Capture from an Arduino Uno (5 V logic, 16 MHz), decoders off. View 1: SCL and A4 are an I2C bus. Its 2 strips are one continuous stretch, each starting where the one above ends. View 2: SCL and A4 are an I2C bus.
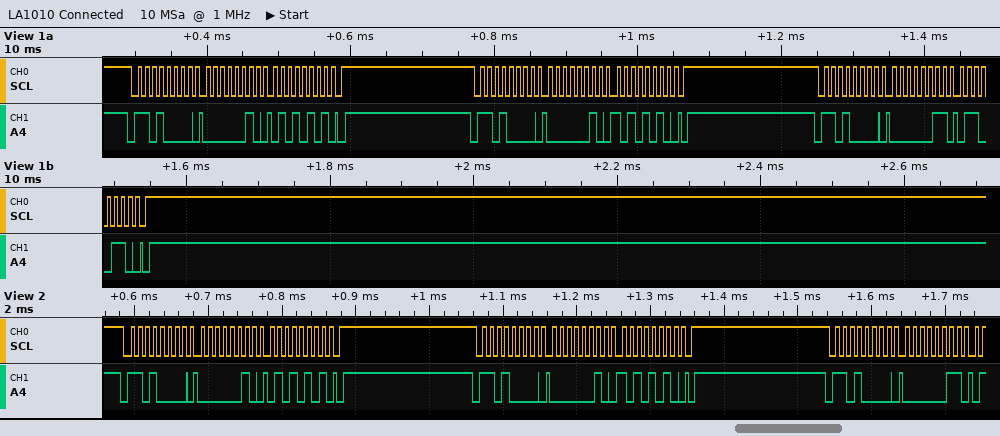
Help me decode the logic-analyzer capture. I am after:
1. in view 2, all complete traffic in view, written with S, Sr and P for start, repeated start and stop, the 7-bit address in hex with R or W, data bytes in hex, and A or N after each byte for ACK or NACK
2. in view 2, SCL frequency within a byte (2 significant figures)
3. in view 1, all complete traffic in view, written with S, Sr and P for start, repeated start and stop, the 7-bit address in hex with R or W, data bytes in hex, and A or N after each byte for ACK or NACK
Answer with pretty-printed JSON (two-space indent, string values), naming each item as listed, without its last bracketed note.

{
  "in view 2, all complete traffic in view, written with S, Sr and P for start, repeated start and stop, the 7-bit address in hex with R or W, data bytes in hex, and A or N after each byte for ACK or NACK": "S 68W A 02 A 55 A P S 68W A 02 A AA A P S 68W A 03 A",
  "in view 2, SCL frequency within a byte": "100 kHz",
  "in view 1, all complete traffic in view, written with S, Sr and P for start, repeated start and stop, the 7-bit address in hex with R or W, data bytes in hex, and A or N after each byte for ACK or NACK": "S 68W A 02 A 55 A P S 68W A 02 A AA A P S 68W A 03 A 66 A P"
}
